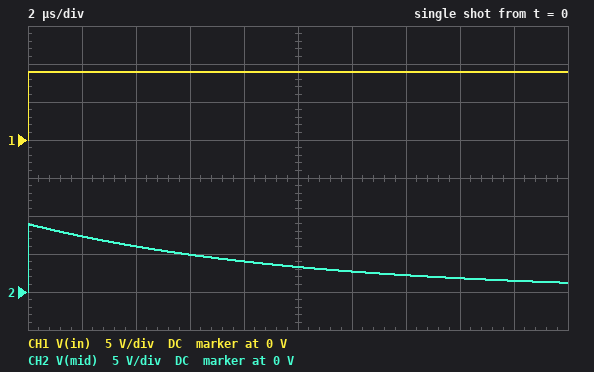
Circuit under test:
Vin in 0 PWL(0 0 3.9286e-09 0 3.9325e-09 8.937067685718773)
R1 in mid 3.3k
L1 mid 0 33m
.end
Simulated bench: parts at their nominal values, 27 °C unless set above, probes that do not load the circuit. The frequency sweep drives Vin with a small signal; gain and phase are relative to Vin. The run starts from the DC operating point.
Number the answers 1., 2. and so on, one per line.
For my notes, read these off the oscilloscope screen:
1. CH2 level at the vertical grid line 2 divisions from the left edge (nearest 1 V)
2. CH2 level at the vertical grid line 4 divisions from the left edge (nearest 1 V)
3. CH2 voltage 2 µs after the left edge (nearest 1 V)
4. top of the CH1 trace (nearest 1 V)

1. 6 V
2. 4 V
3. 7 V
4. 9 V
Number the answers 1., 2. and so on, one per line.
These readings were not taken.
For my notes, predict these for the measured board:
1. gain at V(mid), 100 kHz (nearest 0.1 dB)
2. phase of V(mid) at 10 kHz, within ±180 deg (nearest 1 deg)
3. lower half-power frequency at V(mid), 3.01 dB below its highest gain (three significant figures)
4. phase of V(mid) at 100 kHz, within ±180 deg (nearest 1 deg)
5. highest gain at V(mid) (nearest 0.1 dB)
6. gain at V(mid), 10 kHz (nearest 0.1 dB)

1. -0.1 dB
2. 58 deg
3. 15.9 kHz
4. 9 deg
5. 0 dB
6. -5.5 dB
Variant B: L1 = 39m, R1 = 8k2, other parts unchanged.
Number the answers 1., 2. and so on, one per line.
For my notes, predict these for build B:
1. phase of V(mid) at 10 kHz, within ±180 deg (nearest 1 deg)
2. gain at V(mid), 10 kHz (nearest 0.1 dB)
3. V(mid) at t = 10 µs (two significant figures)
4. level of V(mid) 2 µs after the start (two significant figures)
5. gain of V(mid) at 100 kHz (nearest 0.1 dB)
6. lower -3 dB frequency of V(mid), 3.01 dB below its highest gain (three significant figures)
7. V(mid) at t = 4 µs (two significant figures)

1. 73 deg
2. -10.9 dB
3. 1.1 V
4. 5.9 V
5. -0.5 dB
6. 33.5 kHz
7. 3.9 V
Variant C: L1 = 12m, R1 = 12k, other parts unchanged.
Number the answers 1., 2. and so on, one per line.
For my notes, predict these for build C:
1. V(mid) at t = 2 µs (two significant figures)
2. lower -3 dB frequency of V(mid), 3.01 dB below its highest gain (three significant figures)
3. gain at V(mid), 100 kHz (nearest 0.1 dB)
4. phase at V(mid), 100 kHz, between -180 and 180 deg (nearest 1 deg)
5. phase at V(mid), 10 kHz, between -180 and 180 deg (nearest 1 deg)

1. 1.2 V
2. 159 kHz
3. -5.5 dB
4. 58 deg
5. 86 deg
